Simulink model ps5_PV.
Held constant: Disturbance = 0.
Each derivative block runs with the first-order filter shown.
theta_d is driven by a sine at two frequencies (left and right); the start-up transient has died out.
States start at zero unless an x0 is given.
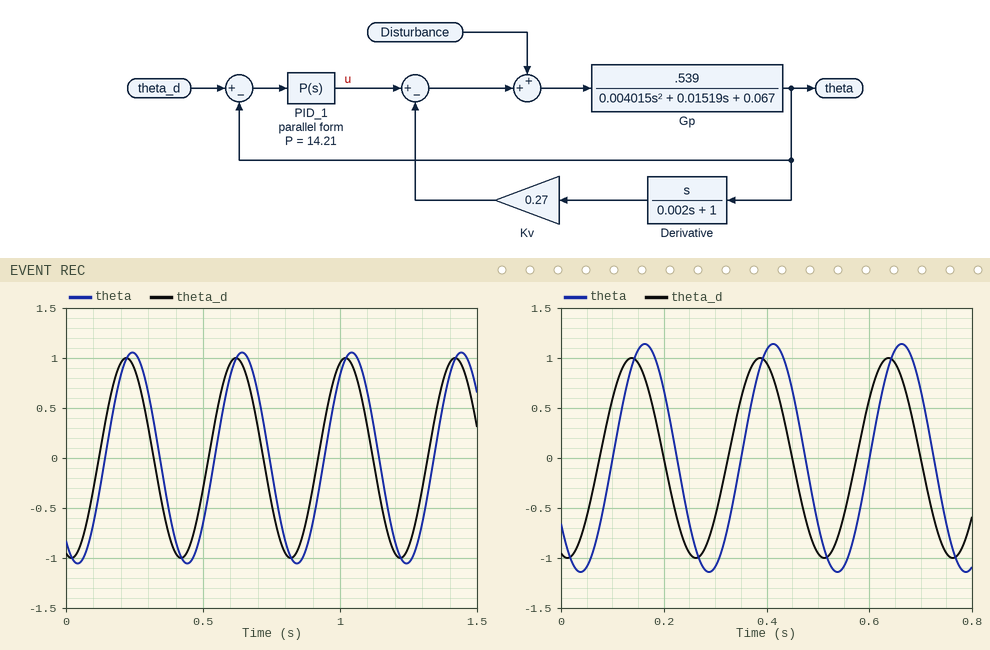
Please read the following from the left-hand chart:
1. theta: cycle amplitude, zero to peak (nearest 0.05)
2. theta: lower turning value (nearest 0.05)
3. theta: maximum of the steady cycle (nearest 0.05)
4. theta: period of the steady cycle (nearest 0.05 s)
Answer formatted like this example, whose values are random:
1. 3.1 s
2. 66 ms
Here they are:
1. 1.05
2. -1.05
3. 1.05
4. 0.40 s
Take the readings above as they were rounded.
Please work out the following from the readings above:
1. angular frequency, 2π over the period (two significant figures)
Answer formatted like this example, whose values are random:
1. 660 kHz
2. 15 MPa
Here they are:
1. 16 rad/s
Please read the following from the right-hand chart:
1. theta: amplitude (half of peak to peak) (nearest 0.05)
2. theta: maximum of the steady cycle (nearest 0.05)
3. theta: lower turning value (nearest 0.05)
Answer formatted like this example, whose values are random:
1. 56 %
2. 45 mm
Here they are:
1. 1.15
2. 1.15
3. -1.15
